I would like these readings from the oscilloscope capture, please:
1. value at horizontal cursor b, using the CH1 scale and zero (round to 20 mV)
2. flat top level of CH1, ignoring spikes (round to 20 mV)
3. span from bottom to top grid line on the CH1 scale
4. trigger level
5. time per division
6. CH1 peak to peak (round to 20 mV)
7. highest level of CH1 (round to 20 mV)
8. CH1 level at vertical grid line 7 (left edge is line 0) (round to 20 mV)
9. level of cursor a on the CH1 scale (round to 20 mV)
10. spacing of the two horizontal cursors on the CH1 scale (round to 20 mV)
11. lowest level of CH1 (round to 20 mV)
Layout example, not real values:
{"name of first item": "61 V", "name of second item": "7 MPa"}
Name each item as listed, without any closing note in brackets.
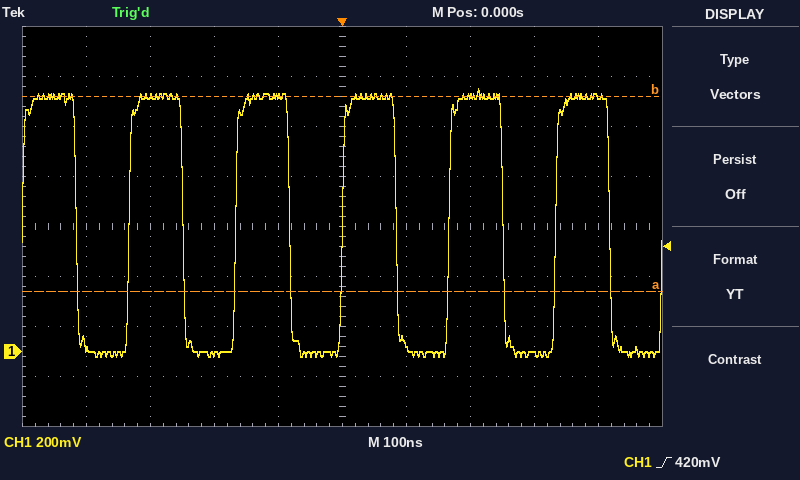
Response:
{"value at horizontal cursor b, using the CH1 scale and zero": "1.02 V", "flat top level of CH1, ignoring spikes": "1.02 V", "span from bottom to top grid line on the CH1 scale": "1.6 V", "trigger level": "420 mV", "time per division": "100 ns", "CH1 peak to peak": "1.08 V", "highest level of CH1": "1.06 V", "CH1 level at vertical grid line 7 (left edge is line 0)": "1.02 V", "level of cursor a on the CH1 scale": "240 mV", "spacing of the two horizontal cursors on the CH1 scale": "780 mV", "lowest level of CH1": "-20 mV"}
